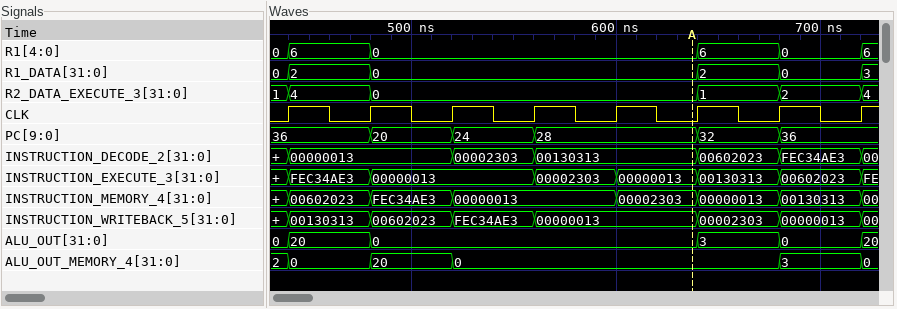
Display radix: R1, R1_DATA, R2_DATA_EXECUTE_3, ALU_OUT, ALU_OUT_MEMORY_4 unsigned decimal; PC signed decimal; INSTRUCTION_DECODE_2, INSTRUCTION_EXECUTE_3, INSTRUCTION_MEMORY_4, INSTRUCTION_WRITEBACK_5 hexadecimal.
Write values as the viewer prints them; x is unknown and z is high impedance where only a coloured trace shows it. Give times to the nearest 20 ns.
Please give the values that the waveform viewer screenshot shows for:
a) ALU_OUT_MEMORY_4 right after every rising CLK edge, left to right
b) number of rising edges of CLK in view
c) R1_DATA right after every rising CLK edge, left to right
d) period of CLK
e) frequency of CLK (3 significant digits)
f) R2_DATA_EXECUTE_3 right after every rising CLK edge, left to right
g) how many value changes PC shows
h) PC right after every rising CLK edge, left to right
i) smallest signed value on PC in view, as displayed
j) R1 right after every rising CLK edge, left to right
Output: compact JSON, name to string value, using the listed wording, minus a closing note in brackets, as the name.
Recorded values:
{"ALU_OUT_MEMORY_4 right after every rising CLK edge, left to right": "0, 20, 0, 0, 0, 0, 3, 0", "number of rising edges of CLK in view": "8", "R1_DATA right after every rising CLK edge, left to right": "2, 0, 0, 0, 0, 2, 0, 3", "period of CLK": "40 ns", "frequency of CLK": "25.0 MHz", "R2_DATA_EXECUTE_3 right after every rising CLK edge, left to right": "4, 0, 0, 0, 0, 1, 2, 4", "how many value changes PC shows": "5", "PC right after every rising CLK edge, left to right": "36, 20, 24, 28, 28, 32, 36, 36", "smallest signed value on PC in view, as displayed": "20", "R1 right after every rising CLK edge, left to right": "6, 0, 0, 0, 0, 6, 0, 6"}
